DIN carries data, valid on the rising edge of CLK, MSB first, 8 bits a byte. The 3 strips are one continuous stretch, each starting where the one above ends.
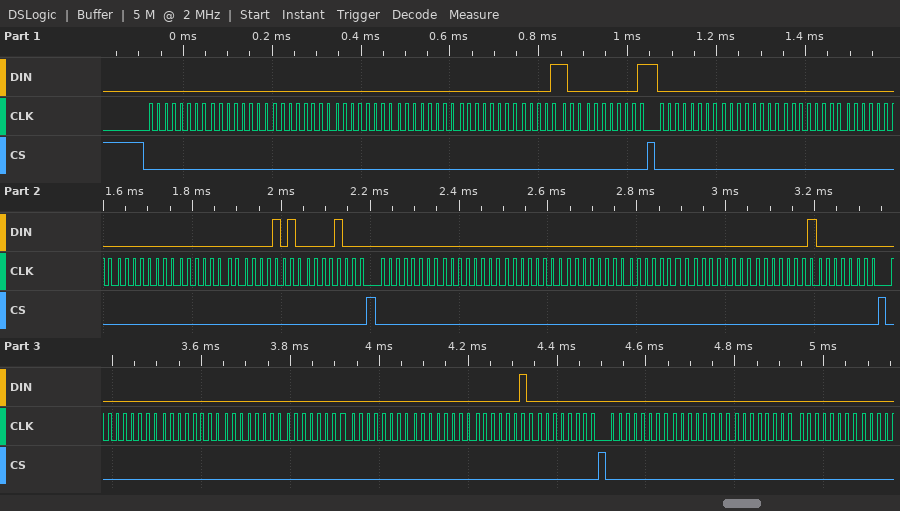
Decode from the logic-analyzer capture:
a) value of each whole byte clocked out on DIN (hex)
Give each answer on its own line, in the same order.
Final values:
0x00 0x00 0x00 0x00 0x00 0x00 0x0C 0x01 0x00 0x00 0x00 0x00 0x00 0x00 0x0A 0x08 0x00 0x00 0x00 0x00 0x00 0x00 0x01 0x00 0x00 0x00 0x00 0x00 0x00 0x00 0x02 0x00 0x00 0x00 0x00 0x00
